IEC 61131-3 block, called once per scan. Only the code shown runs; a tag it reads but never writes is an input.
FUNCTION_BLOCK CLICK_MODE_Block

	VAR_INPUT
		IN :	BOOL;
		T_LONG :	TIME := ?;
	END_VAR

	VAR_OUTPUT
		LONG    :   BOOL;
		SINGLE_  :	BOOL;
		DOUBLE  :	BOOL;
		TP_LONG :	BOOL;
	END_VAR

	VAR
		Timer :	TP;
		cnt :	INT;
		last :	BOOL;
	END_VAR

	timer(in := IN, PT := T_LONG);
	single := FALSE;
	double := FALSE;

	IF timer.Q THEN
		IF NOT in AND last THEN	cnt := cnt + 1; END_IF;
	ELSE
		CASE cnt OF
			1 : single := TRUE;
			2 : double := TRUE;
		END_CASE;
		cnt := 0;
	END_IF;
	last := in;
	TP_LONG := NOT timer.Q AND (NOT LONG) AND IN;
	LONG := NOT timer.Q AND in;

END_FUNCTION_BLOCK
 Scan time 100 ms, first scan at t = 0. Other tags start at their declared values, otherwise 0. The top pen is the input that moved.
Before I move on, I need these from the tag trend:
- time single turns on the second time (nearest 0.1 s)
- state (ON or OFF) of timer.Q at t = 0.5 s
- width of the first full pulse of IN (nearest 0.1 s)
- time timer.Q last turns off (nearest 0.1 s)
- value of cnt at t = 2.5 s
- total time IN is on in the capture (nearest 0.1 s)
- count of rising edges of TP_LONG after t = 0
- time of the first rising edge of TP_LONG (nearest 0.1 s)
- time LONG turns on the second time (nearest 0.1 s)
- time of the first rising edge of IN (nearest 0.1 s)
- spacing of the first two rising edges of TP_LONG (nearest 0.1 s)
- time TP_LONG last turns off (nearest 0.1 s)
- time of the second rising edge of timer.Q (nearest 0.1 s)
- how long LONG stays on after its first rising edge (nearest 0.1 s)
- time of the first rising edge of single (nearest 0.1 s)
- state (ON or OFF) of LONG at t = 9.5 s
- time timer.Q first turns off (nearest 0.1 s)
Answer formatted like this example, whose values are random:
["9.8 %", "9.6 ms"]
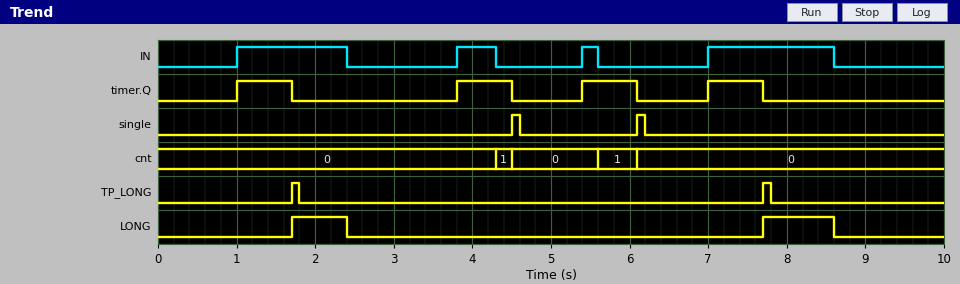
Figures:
["6.1 s", "OFF", "1.4 s", "7.7 s", "0", "3.7 s", "2", "1.7 s", "7.7 s", "1.0 s", "6.0 s", "7.8 s", "3.8 s", "0.7 s", "4.5 s", "OFF", "1.7 s"]
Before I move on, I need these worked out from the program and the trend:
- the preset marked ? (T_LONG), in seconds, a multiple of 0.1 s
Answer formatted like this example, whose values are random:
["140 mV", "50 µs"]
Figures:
["0.7 s"]
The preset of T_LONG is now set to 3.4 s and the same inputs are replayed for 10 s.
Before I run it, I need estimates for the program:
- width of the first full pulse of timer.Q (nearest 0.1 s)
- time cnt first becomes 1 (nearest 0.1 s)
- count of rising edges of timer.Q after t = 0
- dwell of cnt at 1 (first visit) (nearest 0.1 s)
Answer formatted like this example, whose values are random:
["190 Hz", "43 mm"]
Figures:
["3.4 s", "2.4 s", "2", "1.9 s"]
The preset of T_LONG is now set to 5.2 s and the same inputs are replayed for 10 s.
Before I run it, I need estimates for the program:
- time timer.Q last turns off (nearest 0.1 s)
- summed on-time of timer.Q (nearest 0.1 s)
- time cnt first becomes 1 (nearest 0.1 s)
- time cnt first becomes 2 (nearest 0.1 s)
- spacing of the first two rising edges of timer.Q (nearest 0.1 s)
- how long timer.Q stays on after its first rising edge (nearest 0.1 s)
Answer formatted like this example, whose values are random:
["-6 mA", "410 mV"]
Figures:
["6.2 s", "8.2 s", "2.4 s", "4.3 s", "6.0 s", "5.2 s"]
